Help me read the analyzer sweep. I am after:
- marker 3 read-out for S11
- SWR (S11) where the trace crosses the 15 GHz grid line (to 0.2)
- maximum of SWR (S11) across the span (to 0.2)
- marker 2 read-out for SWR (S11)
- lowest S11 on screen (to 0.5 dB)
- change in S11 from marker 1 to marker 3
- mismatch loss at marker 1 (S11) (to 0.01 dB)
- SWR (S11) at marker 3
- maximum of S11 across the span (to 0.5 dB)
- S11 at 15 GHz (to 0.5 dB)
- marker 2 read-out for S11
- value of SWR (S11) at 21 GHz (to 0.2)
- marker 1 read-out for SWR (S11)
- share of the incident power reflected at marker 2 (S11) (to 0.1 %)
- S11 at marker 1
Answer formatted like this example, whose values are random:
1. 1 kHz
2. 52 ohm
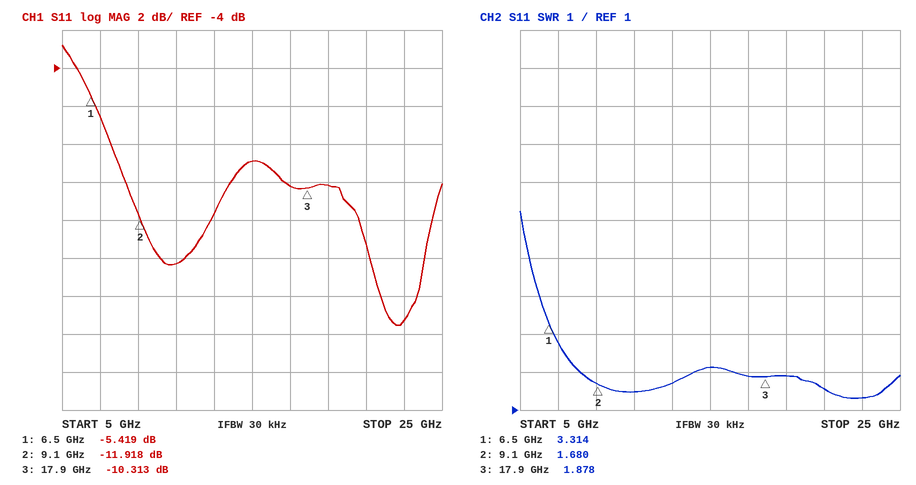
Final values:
1. -10.313 dB
2. 2.2
3. 6.2
4. 1.680
5. -17.5 dB
6. -4.894 dB
7. 1.47 dB
8. 1.878
9. -3.0 dB
10. -9.0 dB
11. -11.918 dB
12. 1.6
13. 3.314
14. 6.4 %
15. -5.419 dB
